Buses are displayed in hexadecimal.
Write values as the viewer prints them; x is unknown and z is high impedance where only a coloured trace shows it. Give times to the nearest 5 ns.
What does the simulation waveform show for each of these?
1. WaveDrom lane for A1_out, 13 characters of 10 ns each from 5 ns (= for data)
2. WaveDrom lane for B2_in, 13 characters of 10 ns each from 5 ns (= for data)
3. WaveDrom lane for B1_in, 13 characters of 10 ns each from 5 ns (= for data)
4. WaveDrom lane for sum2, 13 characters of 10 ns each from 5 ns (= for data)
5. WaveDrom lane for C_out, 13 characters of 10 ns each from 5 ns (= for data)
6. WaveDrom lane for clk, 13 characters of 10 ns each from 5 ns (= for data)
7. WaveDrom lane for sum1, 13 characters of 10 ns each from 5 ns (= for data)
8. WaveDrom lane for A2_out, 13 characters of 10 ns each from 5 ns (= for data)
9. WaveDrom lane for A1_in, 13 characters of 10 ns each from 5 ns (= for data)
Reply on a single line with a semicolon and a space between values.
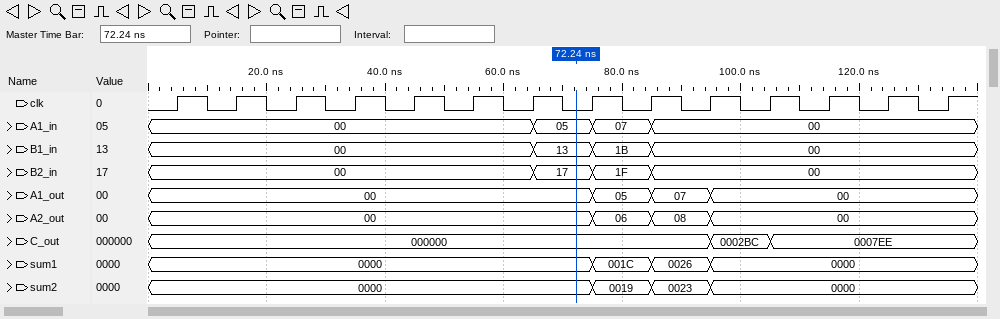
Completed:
{name: 'A1_out', wave: '=......===...', data: '00 05 07 00'}; {name: 'B2_in', wave: '=.....===....', data: '00 17 1F 00'}; {name: 'B1_in', wave: '=.....===....', data: '00 13 1B 00'}; {name: 'sum2', wave: '=......===...', data: '0000 0019 0023 0000'}; {name: 'C_out', wave: '=........==..', data: '000000 0002BC 0007EE'}; {name: 'clk', wave: 'p............'}; {name: 'sum1', wave: '=......===...', data: '0000 001C 0026 0000'}; {name: 'A2_out', wave: '=......===...', data: '00 06 08 00'}; {name: 'A1_in', wave: '=.....===....', data: '00 05 07 00'}
